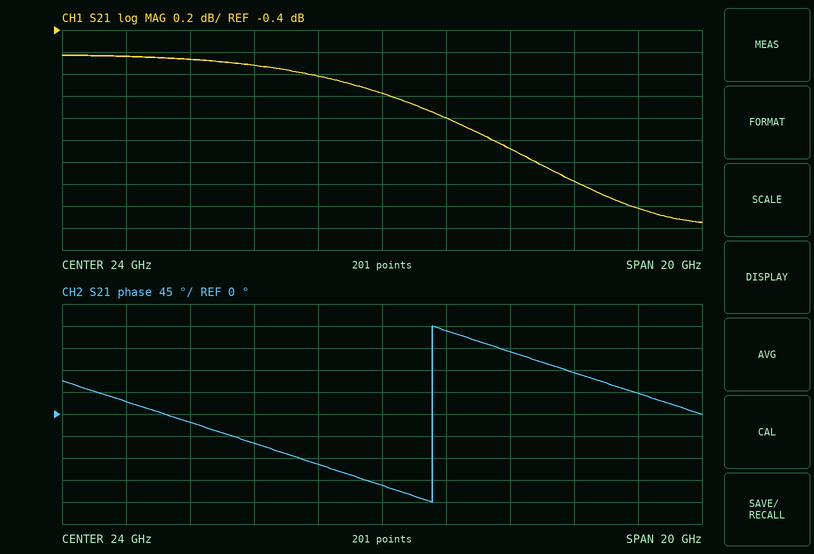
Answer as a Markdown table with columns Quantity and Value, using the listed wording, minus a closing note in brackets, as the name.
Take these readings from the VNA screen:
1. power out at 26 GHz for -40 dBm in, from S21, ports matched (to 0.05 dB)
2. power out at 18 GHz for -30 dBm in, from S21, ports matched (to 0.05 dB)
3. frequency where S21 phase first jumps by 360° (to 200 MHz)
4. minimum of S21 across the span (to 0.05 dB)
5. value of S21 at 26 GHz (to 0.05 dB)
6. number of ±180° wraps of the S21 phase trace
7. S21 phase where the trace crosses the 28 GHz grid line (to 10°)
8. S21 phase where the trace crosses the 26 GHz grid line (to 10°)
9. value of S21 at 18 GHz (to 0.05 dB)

| Quantity | Value |
|---|---|
| power out at 26 GHz for -40 dBm in, from S21, ports matched | -41.20 dBm |
| power out at 18 GHz for -30 dBm in, from S21, ports matched | -30.65 dBm |
| frequency where S21 phase first jumps by 360° | 25.6 GHz |
| minimum of S21 across the span | -2.15 dB |
| value of S21 at 26 GHz | -1.20 dB |
| number of ±180° wraps of the S21 phase trace | 1 |
| S21 phase where the trace crosses the 28 GHz grid line | 130° |
| S21 phase where the trace crosses the 26 GHz grid line | 170° |
| value of S21 at 18 GHz | -0.65 dB |
